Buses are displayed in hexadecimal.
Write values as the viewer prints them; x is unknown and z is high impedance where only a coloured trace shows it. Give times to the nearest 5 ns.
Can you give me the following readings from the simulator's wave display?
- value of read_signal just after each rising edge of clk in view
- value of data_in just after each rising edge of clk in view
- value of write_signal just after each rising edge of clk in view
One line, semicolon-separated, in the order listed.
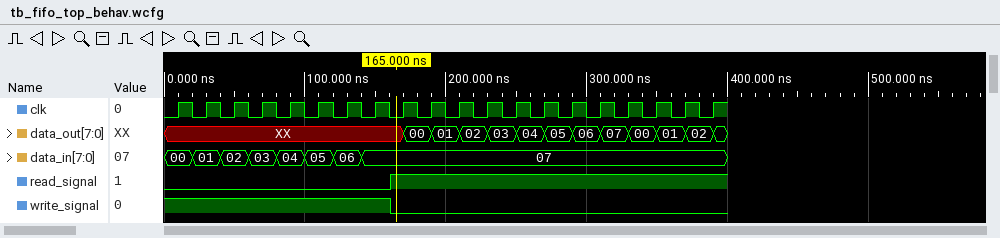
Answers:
0 0 0 0 0 0 0 0 1 1 1 1 1 1 1 1 1 1 1 1; 00, 01, 02, 03, 04, 05, 06, 07, 07, 07, 07, 07, 07, 07, 07, 07, 07, 07, 07, 07; 1 1 1 1 1 1 1 1 0 0 0 0 0 0 0 0 0 0 0 0
